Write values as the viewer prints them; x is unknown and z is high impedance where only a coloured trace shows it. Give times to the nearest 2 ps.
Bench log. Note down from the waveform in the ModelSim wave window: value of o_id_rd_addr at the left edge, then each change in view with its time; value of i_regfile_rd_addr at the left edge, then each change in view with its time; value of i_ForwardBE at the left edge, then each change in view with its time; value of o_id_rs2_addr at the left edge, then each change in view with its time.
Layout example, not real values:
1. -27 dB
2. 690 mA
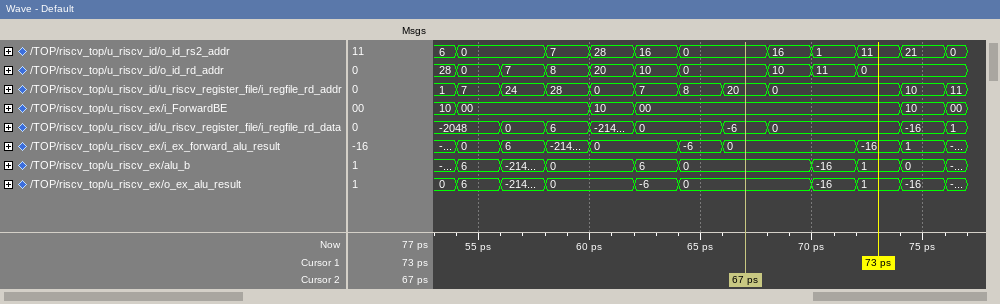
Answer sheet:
1. 28, 0 at 54 ps, 7 at 56 ps, 8 at 58 ps, 20 at 60 ps, 10 at 62 ps, 0 at 64 ps, 10 at 68 ps, 11 at 70 ps, 0 at 72 ps
2. 1, 7 at 54 ps, 24 at 56 ps, 28 at 58 ps, 0 at 60 ps, 7 at 62 ps, 8 at 64 ps, 20 at 66 ps, 0 at 68 ps, 10 at 74 ps, 11 at 76 ps
3. 10, 00 at 54 ps, 10 at 60 ps, 00 at 62 ps, 10 at 74 ps, 00 at 76 ps
4. 6, 0 at 54 ps, 7 at 58 ps, 28 at 60 ps, 16 at 62 ps, 0 at 64 ps, 16 at 68 ps, 1 at 70 ps, 11 at 72 ps, 21 at 74 ps, 0 at 76 ps
